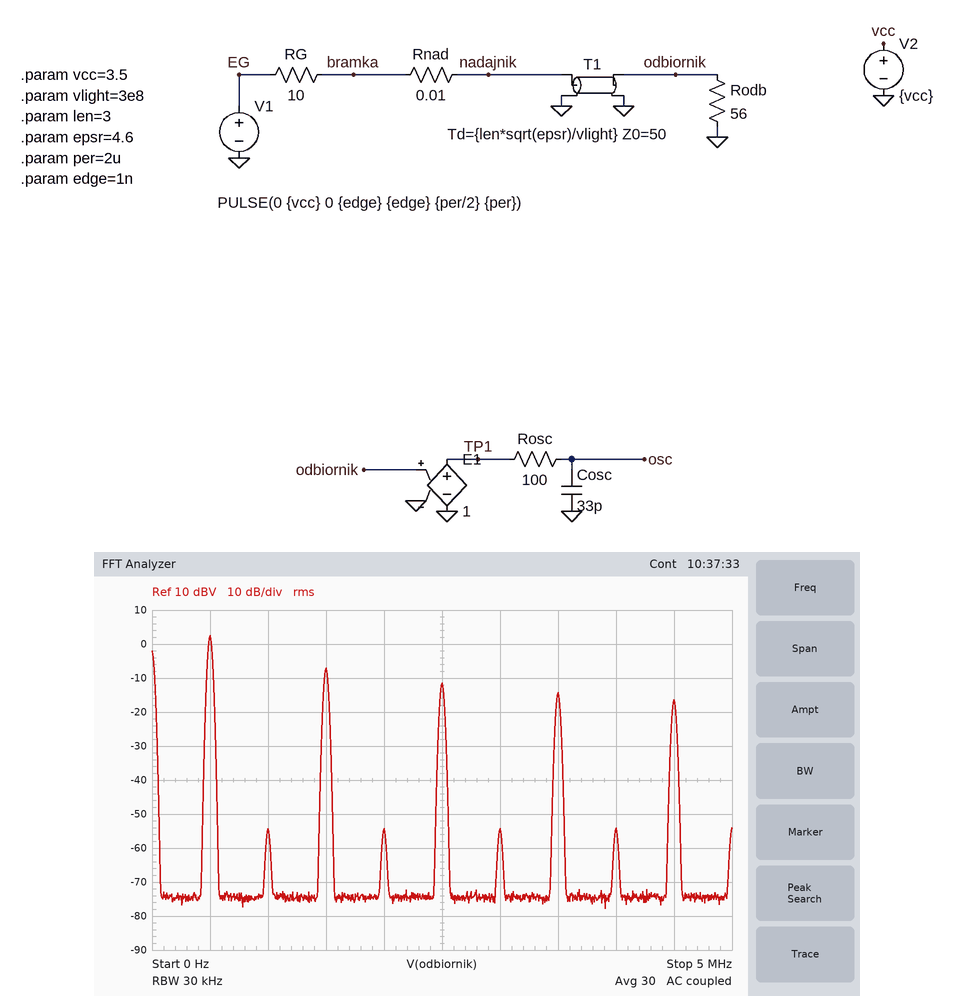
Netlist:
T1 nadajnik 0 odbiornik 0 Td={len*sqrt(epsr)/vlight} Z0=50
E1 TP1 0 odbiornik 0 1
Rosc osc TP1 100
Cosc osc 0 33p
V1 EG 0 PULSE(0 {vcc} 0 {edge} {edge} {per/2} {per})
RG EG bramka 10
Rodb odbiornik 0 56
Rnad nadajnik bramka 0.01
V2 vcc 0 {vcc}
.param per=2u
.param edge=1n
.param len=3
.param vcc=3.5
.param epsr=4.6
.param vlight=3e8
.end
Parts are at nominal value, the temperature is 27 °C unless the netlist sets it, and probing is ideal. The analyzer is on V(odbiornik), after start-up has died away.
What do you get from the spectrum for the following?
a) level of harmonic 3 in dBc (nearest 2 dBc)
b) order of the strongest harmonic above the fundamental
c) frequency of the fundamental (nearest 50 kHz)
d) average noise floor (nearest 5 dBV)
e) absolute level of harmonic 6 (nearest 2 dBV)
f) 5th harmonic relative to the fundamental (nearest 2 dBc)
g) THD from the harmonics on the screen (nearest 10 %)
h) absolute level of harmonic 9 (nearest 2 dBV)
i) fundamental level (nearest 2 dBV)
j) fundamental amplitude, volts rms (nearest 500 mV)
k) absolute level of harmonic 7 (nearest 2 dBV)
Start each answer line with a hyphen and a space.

- -10 dBc
- 3
- 500 kHz
- -75 dBV
- -54 dBV
- -14 dBc
- 40 %
- -16 dBV
- 2 dBV
- 1.5 V
- -14 dBV
